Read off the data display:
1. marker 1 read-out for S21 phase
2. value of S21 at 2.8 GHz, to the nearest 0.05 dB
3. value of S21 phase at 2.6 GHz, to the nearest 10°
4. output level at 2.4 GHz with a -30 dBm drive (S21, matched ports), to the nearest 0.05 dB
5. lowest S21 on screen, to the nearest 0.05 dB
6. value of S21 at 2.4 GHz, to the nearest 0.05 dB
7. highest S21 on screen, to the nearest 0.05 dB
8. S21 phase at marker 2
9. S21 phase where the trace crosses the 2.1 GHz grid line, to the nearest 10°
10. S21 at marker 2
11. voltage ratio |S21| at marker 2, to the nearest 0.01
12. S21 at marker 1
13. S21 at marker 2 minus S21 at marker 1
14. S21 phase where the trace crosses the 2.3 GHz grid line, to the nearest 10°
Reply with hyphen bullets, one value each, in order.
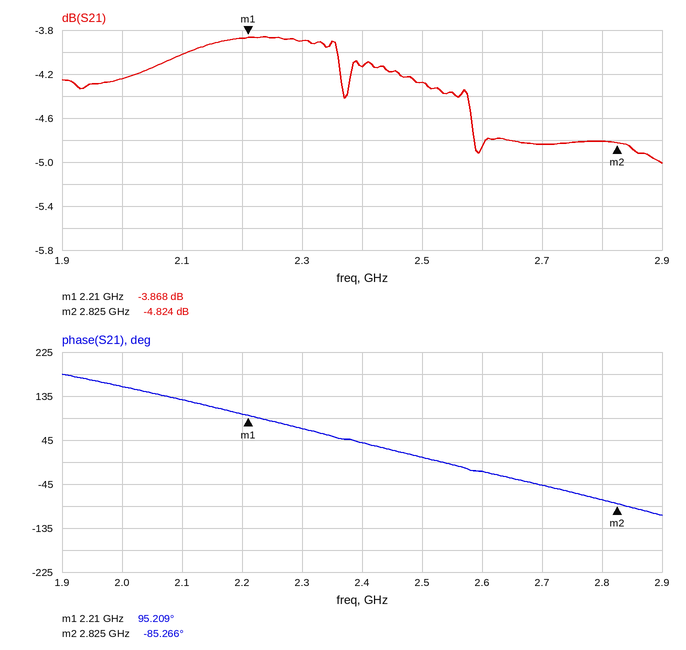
- 95.209°
- -4.80 dB
- -20°
- -34.15 dBm
- -5.00 dB
- -4.15 dB
- -3.85 dB
- -85.266°
- 130°
- -4.824 dB
- 0.57
- -3.868 dB
- -0.956 dB
- 70°
